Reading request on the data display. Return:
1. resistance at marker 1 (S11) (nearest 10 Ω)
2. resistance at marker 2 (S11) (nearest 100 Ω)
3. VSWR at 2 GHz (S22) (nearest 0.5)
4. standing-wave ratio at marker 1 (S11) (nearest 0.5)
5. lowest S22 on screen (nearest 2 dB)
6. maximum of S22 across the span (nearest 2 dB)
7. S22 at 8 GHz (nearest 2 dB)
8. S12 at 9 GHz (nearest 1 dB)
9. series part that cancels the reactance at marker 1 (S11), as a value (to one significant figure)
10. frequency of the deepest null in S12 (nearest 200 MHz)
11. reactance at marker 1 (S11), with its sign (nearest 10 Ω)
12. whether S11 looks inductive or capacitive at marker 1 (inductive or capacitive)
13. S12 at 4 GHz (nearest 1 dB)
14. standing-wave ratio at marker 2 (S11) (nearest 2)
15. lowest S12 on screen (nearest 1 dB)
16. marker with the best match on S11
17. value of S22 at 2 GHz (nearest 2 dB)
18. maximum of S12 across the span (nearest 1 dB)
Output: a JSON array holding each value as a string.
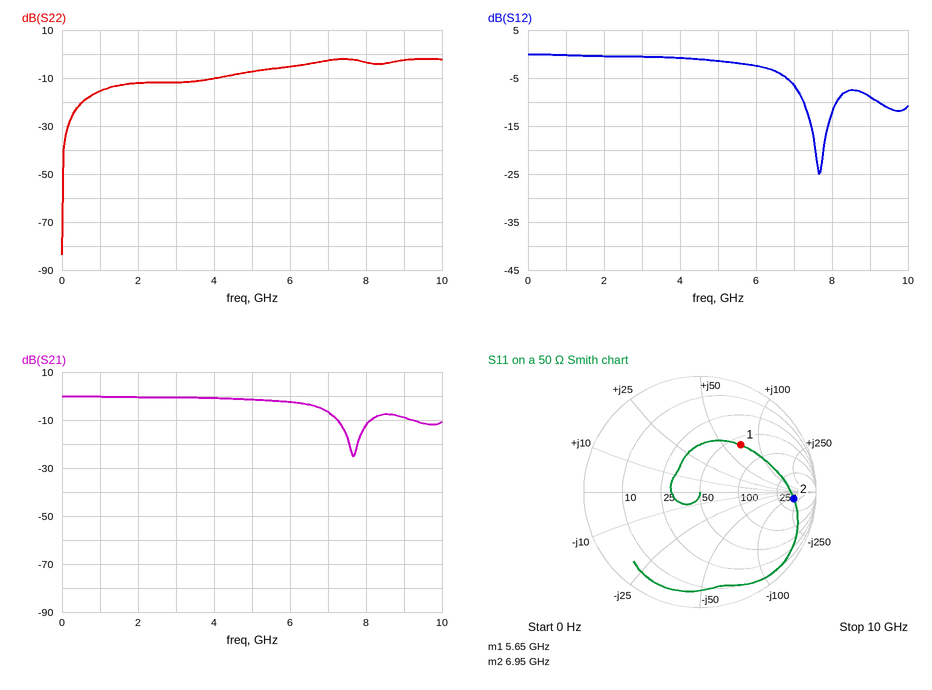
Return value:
["60 Ω", "400 Ω", "1.5", "3.5", "-84 dB", "-2 dB", "-4 dB", "-9 dB", "400 fF", "7.6 GHz", "+70 Ω", "inductive", "-1 dB", "10", "-25 dB", "marker 1", "-12 dB", "0 dB"]
